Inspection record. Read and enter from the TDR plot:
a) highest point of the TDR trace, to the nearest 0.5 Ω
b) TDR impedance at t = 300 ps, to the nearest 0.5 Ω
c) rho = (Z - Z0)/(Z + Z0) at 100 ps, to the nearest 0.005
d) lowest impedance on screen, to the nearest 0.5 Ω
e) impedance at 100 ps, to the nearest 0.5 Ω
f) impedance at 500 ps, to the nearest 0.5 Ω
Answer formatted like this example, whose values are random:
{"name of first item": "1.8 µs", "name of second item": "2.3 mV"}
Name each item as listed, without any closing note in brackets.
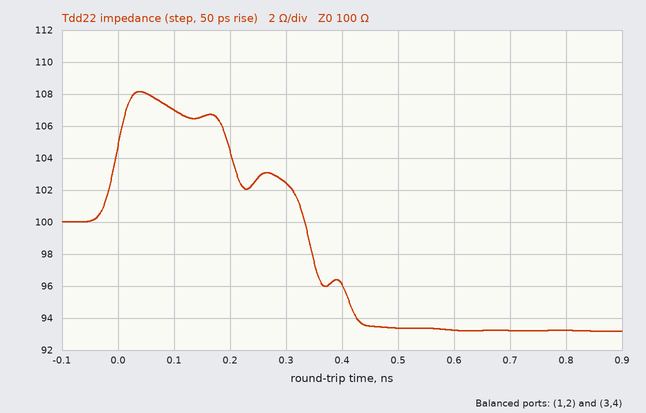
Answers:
{"highest point of the TDR trace, to the nearest 0.5 Ω": "108.0 Ω", "TDR impedance at t = 300 ps, to the nearest 0.5 Ω": "102.5 Ω", "rho = (Z - Z0)/(Z + Z0) at 100 ps, to the nearest 0.005": "+0.035", "lowest impedance on screen, to the nearest 0.5 Ω": "93.0 Ω", "impedance at 100 ps, to the nearest 0.5 Ω": "107.0 Ω", "impedance at 500 ps, to the nearest 0.5 Ω": "93.5 Ω"}
